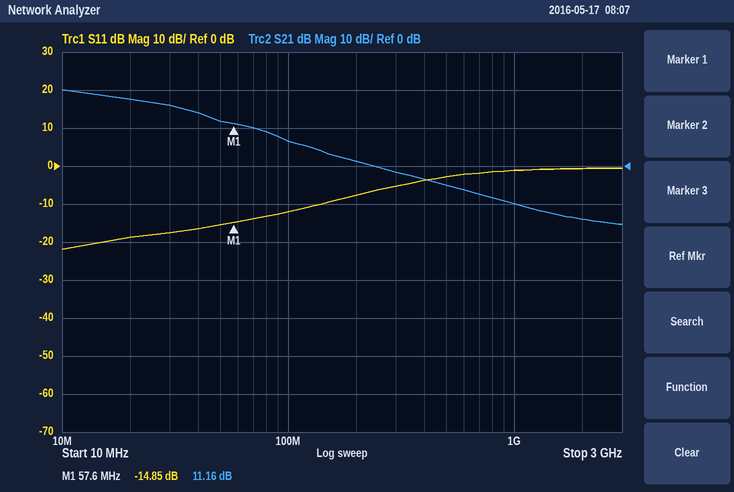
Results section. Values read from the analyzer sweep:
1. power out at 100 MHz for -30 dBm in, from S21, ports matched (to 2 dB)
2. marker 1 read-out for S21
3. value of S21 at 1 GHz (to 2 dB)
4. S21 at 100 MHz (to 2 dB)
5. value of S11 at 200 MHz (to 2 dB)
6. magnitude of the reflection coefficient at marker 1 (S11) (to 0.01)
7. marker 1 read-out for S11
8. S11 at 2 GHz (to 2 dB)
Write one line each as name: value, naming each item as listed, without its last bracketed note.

power out at 100 MHz for -30 dBm in, from S21, ports matched: -24 dBm
marker 1 read-out for S21: 11.16 dB
value of S21 at 1 GHz: -10 dB
S21 at 100 MHz: 6 dB
value of S11 at 200 MHz: -8 dB
magnitude of the reflection coefficient at marker 1 (S11): 0.18
marker 1 read-out for S11: -14.85 dB
S11 at 2 GHz: 0 dB
